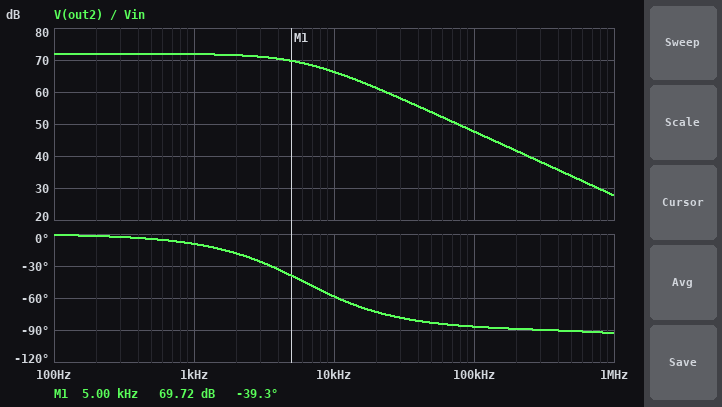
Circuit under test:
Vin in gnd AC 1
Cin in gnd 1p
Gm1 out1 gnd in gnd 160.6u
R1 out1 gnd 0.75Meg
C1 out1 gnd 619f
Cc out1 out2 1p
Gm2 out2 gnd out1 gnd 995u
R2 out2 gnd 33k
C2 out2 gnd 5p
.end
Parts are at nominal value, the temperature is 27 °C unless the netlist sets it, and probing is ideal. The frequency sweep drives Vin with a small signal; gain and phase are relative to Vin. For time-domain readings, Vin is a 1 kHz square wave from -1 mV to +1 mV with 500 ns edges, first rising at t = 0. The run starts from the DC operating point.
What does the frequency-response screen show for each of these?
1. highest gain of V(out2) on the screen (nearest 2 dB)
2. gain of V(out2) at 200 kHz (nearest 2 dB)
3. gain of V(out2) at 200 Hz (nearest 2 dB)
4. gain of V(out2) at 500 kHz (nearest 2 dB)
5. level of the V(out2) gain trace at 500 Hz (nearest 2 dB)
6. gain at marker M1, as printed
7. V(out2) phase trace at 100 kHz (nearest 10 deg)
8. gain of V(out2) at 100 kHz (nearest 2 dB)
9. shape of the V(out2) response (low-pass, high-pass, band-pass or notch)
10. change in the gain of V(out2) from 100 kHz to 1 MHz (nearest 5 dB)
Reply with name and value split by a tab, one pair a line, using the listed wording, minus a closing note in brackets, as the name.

highest gain of V(out2) on the screen	72 dB
gain of V(out2) at 200 kHz	42 dB
gain of V(out2) at 200 Hz	72 dB
gain of V(out2) at 500 kHz	34 dB
level of the V(out2) gain trace at 500 Hz	72 dB
gain at marker M1, as printed	69.72 dB
V(out2) phase trace at 100 kHz	-90 deg
gain of V(out2) at 100 kHz	48 dB
shape of the V(out2) response	low-pass
change in the gain of V(out2) from 100 kHz to 1 MHz	-20 dB
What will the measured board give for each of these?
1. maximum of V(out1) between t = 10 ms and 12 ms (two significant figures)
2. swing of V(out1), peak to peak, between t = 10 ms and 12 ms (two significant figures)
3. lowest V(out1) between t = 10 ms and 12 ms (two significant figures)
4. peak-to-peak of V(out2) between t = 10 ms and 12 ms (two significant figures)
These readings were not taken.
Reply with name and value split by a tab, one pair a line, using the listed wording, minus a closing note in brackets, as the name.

maximum of V(out1) between t = 10 ms and 12 ms	120 mV
swing of V(out1), peak to peak, between t = 10 ms and 12 ms	240 mV
lowest V(out1) between t = 10 ms and 12 ms	-120 mV
peak-to-peak of V(out2) between t = 10 ms and 12 ms	7.9 V
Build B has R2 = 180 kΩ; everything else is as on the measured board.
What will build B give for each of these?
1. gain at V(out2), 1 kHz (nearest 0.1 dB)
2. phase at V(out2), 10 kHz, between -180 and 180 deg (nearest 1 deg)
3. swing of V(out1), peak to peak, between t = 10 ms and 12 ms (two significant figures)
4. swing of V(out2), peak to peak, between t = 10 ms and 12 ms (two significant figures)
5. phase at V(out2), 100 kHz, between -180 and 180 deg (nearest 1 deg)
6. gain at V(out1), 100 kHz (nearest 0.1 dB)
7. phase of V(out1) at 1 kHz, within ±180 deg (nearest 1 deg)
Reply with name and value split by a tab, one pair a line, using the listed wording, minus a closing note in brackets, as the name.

gain at V(out2), 1 kHz	84.3 dB
phase at V(out2), 10 kHz, between -180 and 180 deg	-83 deg
swing of V(out1), peak to peak, between t = 10 ms and 12 ms	230 mV
swing of V(out2), peak to peak, between t = 10 ms and 12 ms	41 V
phase at V(out2), 100 kHz, between -180 and 180 deg	-90 deg
gain at V(out1), 100 kHz	4.6 dB
phase of V(out1) at 1 kHz, within ±180 deg	140 deg
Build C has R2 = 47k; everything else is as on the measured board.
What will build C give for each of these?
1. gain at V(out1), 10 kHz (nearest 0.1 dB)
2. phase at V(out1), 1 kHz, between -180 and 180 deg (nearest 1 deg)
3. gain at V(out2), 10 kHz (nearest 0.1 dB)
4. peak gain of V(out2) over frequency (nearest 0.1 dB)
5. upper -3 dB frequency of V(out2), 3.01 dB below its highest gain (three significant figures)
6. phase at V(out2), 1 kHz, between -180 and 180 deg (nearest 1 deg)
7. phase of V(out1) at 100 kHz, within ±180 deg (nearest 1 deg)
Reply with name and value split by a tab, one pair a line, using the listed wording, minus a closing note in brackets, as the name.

gain at V(out1), 10 kHz	33.6 dB
phase at V(out1), 1 kHz, between -180 and 180 deg	167 deg
gain at V(out2), 10 kHz	67.0 dB
peak gain of V(out2) over frequency	75.0 dB
upper -3 dB frequency of V(out2), 3.01 dB below its highest gain	4.35 kHz
phase at V(out2), 1 kHz, between -180 and 180 deg	-13 deg
phase of V(out1) at 100 kHz, within ±180 deg	102 deg
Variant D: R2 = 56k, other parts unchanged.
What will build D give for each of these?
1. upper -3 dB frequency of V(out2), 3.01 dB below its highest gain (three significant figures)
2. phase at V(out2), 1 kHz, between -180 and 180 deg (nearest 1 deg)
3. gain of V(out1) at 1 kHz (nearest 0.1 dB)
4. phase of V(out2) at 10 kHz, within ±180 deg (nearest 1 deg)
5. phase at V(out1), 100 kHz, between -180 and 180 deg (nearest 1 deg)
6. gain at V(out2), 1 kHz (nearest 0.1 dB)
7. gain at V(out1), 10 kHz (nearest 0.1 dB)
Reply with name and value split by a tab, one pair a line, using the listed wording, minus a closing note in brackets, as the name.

upper -3 dB frequency of V(out2), 3.01 dB below its highest gain	3.67 kHz
phase at V(out2), 1 kHz, between -180 and 180 deg	-15 deg
gain of V(out1) at 1 kHz	41.3 dB
phase of V(out2) at 10 kHz, within ±180 deg	-70 deg
phase at V(out1), 100 kHz, between -180 and 180 deg	104 deg
gain at V(out2), 1 kHz	76.2 dB
gain at V(out1), 10 kHz	32.4 dB
